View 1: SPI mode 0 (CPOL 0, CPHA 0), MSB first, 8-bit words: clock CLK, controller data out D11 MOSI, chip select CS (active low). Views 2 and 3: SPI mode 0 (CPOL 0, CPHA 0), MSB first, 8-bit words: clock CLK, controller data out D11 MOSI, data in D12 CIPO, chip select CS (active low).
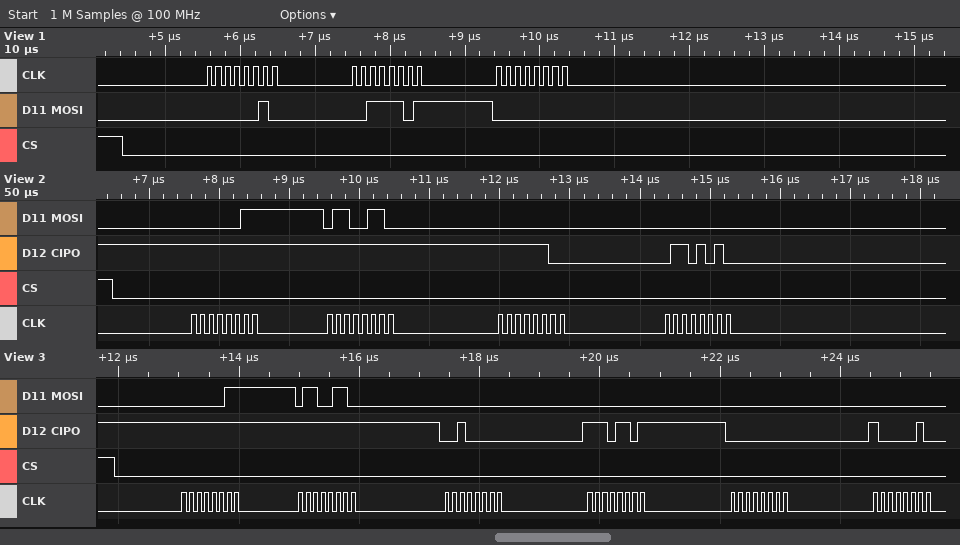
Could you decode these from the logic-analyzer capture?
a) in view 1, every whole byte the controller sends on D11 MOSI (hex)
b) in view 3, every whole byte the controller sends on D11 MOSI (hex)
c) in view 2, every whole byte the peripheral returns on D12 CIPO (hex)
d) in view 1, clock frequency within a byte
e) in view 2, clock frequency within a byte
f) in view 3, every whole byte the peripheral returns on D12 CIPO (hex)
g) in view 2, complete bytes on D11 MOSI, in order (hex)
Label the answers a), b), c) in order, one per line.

a) 02 3D 00
b) 03 66 00 00 00 00
c) FF FF FC 6A
d) 8 MHz
e) 8 MHz
f) FF FF 20 ED 00 82
g) 03 66 00 00
